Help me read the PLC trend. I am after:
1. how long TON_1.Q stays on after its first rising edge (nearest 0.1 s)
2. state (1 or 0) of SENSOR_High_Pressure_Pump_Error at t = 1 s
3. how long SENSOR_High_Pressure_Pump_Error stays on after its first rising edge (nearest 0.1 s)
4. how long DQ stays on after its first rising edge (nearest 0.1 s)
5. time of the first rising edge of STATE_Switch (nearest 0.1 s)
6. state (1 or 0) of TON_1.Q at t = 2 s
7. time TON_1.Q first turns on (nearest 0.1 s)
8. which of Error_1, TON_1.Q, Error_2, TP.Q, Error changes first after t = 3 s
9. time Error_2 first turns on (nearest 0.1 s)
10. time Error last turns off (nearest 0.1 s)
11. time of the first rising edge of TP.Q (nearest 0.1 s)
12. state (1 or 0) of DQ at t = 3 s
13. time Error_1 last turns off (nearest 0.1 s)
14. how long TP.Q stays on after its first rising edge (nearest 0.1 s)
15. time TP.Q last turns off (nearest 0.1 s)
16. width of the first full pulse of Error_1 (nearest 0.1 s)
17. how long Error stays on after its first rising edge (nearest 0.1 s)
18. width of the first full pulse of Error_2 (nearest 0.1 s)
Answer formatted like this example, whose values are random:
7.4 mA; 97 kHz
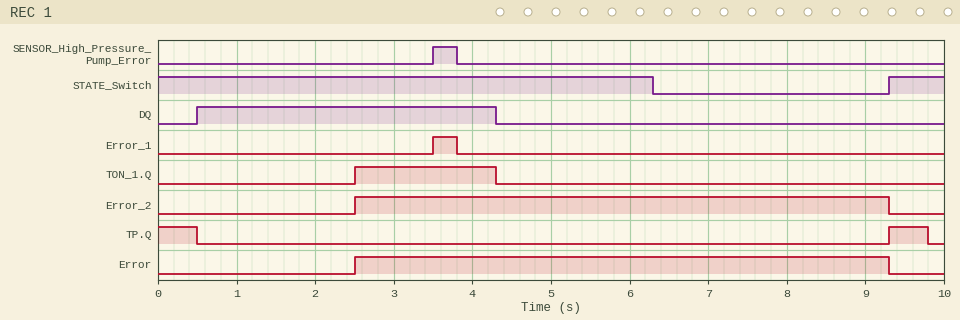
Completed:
1.8 s; 0; 0.3 s; 3.8 s; 9.3 s; 0; 2.5 s; Error_1; 2.5 s; 9.3 s; 9.3 s; 1; 3.8 s; 0.5 s; 9.8 s; 0.3 s; 6.8 s; 6.8 s
